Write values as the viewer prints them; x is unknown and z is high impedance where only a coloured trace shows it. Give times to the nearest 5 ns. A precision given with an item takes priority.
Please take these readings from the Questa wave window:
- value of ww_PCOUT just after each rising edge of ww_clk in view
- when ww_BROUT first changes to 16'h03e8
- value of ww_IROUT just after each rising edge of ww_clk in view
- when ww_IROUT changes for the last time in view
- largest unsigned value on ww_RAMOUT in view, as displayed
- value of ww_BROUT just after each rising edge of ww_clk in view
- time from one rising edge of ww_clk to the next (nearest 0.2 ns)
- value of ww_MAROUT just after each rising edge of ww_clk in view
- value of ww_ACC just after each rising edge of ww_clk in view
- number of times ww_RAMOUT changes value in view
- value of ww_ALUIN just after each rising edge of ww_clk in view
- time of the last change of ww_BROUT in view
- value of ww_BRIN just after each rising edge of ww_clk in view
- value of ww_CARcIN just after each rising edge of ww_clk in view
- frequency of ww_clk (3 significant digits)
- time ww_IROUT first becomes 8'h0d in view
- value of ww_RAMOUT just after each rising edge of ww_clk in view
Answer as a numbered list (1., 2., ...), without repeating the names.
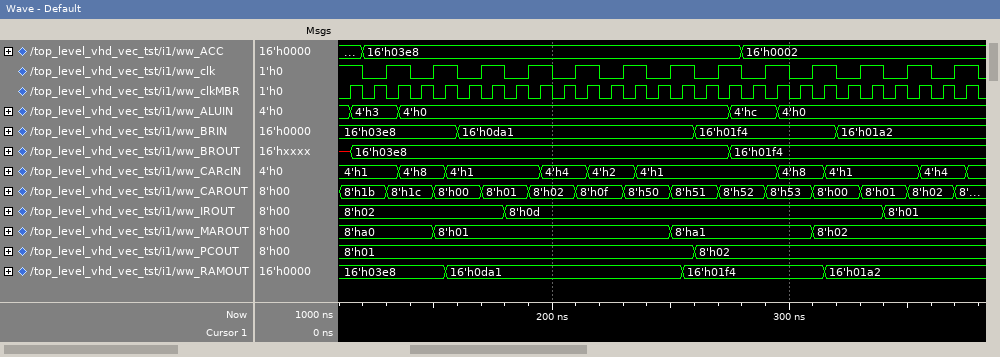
1. 8'h01, 8'h01, 8'h01, 8'h01, 8'h01, 8'h01, 8'h01, 8'h02, 8'h02, 8'h02, 8'h02, 8'h02, 8'h02
2. 115 ns
3. 8'h02, 8'h02, 8'h02, 8'h0d, 8'h0d, 8'h0d, 8'h0d, 8'h0d, 8'h0d, 8'h0d, 8'h0d, 8'h01, 8'h01
4. 340 ns
5. 16'h0da1
6. 16'h03e8, 16'h03e8, 16'h03e8, 16'h03e8, 16'h03e8, 16'h03e8, 16'h03e8, 16'h03e8, 16'h01f4, 16'h01f4, 16'h01f4, 16'h01f4, 16'h01f4
7. 20 ns
8. 8'ha0, 8'h01, 8'h01, 8'h01, 8'h01, 8'h01, 8'ha1, 8'ha1, 8'ha1, 8'h02, 8'h02, 8'h02, 8'h02
9. 16'h03e8, 16'h03e8, 16'h03e8, 16'h03e8, 16'h03e8, 16'h03e8, 16'h03e8, 16'h03e8, 16'h0002, 16'h0002, 16'h0002, 16'h0002, 16'h0002
10. 3
11. 4'h3, 4'h0, 4'h0, 4'h0, 4'h0, 4'h0, 4'h0, 4'h0, 4'hc, 4'h0, 4'h0, 4'h0, 4'h0
12. 275 ns
13. 16'h03e8, 16'h03e8, 16'h0da1, 16'h0da1, 16'h0da1, 16'h0da1, 16'h0da1, 16'h01f4, 16'h01f4, 16'h01f4, 16'h01a2, 16'h01a2, 16'h01a2
14. 4'h1, 4'h8, 4'h1, 4'h1, 4'h4, 4'h2, 4'h1, 4'h1, 4'h1, 4'h8, 4'h1, 4'h1, 4'h4
15. 50.0 MHz
16. 180 ns
17. 16'h03e8, 16'h03e8, 16'h0da1, 16'h0da1, 16'h0da1, 16'h0da1, 16'h0da1, 16'h01f4, 16'h01f4, 16'h01f4, 16'h01a2, 16'h01a2, 16'h01a2
